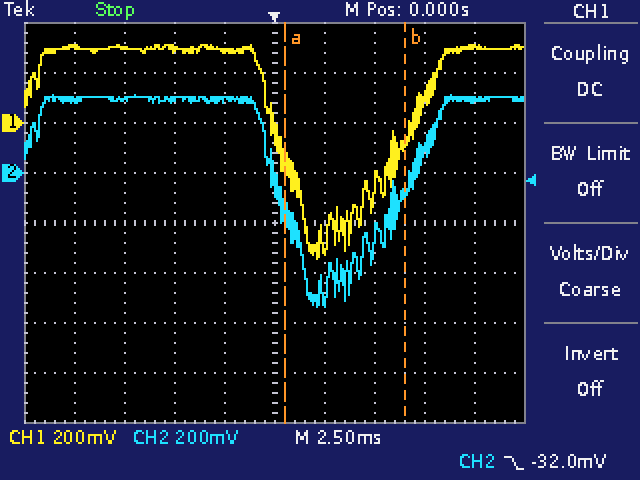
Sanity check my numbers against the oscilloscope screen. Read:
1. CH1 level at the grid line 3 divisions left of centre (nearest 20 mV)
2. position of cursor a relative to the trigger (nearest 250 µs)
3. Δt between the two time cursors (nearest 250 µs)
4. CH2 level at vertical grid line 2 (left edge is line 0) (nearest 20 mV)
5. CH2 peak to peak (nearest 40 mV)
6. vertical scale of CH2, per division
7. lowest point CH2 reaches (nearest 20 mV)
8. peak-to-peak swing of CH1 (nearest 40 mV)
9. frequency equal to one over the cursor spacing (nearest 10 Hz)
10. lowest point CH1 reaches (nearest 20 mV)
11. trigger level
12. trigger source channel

300 mV
+500 µs
6.00 ms
300 mV
840 mV
200 mV
-540 mV
840 mV
170 Hz
-540 mV
-32.0 mV
CH2
